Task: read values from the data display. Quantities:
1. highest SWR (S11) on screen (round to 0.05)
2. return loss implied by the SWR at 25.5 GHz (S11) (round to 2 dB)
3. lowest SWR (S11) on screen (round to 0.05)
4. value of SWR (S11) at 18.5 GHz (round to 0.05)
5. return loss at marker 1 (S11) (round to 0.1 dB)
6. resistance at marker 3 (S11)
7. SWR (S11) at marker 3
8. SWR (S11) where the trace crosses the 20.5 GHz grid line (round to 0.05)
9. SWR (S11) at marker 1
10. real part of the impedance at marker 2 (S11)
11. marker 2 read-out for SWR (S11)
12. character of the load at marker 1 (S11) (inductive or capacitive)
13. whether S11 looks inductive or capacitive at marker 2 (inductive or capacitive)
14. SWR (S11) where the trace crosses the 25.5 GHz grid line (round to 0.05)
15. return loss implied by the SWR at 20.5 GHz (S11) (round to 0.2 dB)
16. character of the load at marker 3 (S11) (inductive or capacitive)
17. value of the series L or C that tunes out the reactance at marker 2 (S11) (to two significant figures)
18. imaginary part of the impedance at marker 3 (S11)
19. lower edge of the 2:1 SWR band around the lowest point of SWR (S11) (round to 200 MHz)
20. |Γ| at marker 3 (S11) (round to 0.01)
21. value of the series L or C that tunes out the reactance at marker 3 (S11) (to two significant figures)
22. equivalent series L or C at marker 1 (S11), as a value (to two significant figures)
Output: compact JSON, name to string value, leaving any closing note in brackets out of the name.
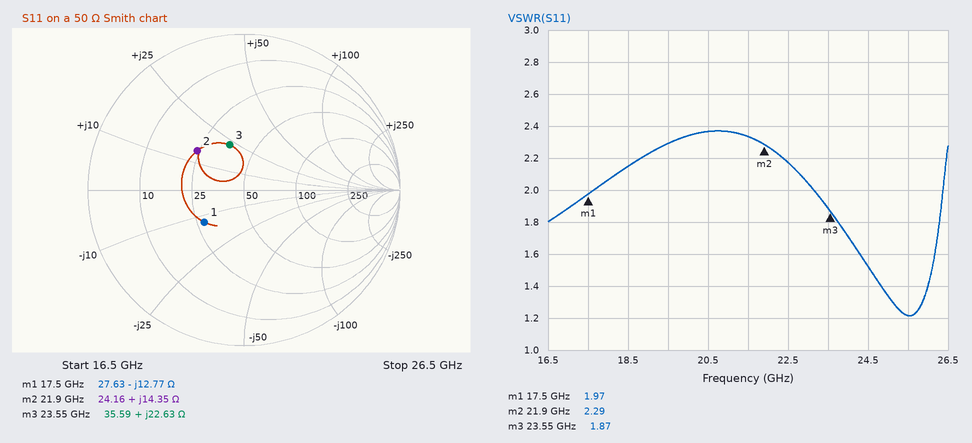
{"highest SWR (S11) on screen": "2.35", "return loss implied by the SWR at 25.5 GHz (S11)": "20 dB", "lowest SWR (S11) on screen": "1.20", "value of SWR (S11) at 18.5 GHz": "2.15", "return loss at marker 1 (S11)": "9.7 dB", "resistance at marker 3": "35.59 Ω", "SWR (S11) at marker 3": "1.87", "SWR (S11) where the trace crosses the 20.5 GHz grid line": "2.35", "SWR (S11) at marker 1": "1.97", "real part of the impedance at marker 2": "24.16 Ω", "marker 2 read-out for SWR": "2.29", "character of the load at marker 1 (S11)": "capacitive", "whether S11 looks inductive or capacitive at marker 2": "inductive", "SWR (S11) where the trace crosses the 25.5 GHz grid line": "1.20", "return loss implied by the SWR at 20.5 GHz (S11)": "7.8 dB", "character of the load at marker 3 (S11)": "inductive", "value of the series L or C that tunes out the reactance at marker 2 (S11)": "510 fF", "imaginary part of the impedance at marker 3": "+22.63 Ω", "lower edge of the 2:1 SWR band around the lowest point of SWR (S11)": "23.2 GHz", "|Γ| at marker 3 (S11)": "0.30", "value of the series L or C that tunes out the reactance at marker 3 (S11)": "300 fF", "equivalent series L or C at marker 1 (S11), as a value": "710 fF"}
